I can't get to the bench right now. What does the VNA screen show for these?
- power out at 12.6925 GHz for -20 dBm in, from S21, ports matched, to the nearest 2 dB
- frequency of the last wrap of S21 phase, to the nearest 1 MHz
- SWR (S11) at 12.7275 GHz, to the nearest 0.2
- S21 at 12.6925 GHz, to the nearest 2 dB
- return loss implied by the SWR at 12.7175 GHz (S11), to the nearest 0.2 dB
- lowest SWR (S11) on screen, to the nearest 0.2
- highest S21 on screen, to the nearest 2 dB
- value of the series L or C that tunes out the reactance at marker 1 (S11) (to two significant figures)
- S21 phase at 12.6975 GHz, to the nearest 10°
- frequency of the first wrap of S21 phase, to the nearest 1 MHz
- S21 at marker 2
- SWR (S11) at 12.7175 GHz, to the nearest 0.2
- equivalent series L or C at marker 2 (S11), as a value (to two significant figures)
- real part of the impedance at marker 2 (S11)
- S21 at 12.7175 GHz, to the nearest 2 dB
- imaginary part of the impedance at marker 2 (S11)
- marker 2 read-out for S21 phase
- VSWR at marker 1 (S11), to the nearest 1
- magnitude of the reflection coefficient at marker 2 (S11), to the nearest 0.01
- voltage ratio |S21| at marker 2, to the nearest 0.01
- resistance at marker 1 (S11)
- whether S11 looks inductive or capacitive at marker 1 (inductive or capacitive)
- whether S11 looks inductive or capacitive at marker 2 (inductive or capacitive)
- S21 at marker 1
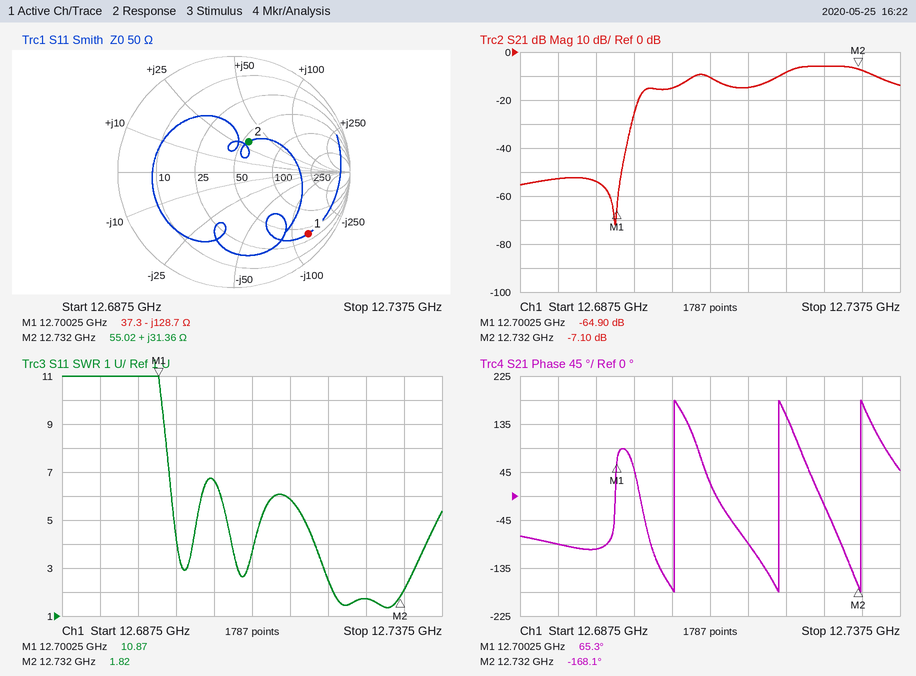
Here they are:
-72 dBm
12.732 GHz
1.8
-52 dB
3.0 dB
1.4
-6 dB
1.6 nH
-100°
12.708 GHz
-7.10 dB
5.8
390 pH
55.02 Ω
-14 dB
+31.36 Ω
-168.1°
11
0.29
0.44
37.3 Ω
capacitive
inductive
-64.90 dB
